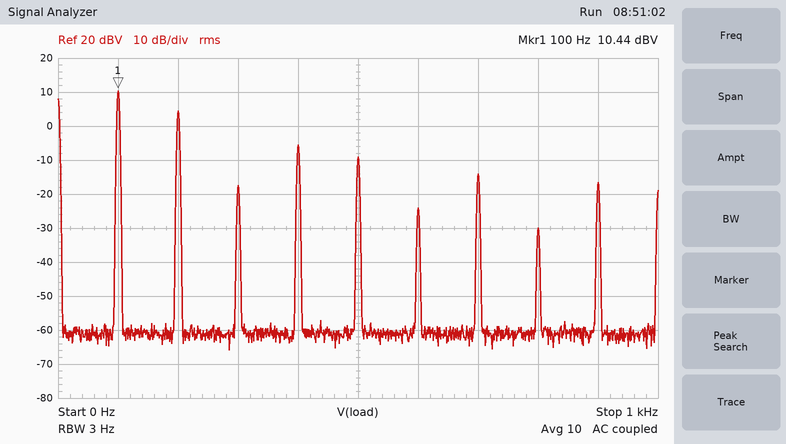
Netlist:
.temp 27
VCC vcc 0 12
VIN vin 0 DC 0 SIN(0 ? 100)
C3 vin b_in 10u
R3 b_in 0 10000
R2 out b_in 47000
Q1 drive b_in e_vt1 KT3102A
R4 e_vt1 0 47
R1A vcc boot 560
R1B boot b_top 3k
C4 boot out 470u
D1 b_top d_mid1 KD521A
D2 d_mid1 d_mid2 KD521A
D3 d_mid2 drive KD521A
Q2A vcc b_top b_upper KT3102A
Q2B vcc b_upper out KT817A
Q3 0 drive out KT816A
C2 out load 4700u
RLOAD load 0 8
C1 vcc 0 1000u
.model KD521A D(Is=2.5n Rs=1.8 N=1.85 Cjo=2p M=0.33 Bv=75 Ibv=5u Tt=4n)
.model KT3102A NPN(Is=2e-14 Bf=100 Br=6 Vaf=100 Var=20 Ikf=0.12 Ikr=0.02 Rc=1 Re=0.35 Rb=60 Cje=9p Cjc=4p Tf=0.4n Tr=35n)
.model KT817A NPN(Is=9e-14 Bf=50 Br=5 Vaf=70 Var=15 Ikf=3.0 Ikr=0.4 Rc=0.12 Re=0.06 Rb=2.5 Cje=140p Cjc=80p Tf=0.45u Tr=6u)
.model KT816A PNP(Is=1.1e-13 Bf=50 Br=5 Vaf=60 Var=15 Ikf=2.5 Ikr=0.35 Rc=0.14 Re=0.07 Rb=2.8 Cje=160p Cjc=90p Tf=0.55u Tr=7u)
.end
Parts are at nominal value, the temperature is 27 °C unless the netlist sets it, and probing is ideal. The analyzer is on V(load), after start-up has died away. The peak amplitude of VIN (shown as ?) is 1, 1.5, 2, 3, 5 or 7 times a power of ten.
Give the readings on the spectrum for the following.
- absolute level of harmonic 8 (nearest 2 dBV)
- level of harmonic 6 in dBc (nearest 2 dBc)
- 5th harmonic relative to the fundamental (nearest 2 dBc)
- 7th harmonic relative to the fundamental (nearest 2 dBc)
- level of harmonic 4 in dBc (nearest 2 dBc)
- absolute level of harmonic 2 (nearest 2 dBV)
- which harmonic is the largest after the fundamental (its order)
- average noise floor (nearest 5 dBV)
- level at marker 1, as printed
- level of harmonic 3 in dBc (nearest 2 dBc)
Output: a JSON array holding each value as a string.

["-30 dBV", "-34 dBc", "-20 dBc", "-24 dBc", "-16 dBc", "4 dBV", "2", "-60 dBV", "10.44 dBV", "-28 dBc"]
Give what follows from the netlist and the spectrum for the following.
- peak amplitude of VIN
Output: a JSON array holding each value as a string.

["2 V"]
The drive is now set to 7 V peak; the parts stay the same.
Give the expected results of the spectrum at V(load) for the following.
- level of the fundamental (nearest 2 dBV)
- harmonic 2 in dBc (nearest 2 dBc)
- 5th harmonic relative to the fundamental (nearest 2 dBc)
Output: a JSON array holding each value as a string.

["8 dBV", "-2 dBc", "-22 dBc"]
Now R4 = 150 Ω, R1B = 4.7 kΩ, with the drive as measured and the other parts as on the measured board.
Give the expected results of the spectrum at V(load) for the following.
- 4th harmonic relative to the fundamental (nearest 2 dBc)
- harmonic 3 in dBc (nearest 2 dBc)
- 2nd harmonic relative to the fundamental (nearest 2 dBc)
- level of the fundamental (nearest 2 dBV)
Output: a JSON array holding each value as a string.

["-40 dBc", "-14 dBc", "-18 dBc", "10 dBV"]
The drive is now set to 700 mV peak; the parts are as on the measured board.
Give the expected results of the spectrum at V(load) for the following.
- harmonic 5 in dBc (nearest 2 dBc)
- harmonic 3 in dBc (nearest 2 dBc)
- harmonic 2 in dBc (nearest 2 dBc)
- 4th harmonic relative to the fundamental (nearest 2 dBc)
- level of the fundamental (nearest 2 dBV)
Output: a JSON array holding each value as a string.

["-22 dBc", "-14 dBc", "-20 dBc", "-28 dBc", "10 dBV"]
